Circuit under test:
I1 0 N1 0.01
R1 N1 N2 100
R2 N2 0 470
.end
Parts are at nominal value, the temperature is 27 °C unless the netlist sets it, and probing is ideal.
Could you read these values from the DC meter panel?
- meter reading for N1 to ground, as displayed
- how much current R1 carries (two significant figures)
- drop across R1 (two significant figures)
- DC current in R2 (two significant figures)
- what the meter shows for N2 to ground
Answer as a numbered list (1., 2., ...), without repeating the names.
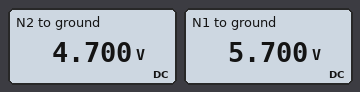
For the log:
1. 5.700 V
2. 10 mA
3. 1.0 V
4. 10 mA
5. 4.700 V
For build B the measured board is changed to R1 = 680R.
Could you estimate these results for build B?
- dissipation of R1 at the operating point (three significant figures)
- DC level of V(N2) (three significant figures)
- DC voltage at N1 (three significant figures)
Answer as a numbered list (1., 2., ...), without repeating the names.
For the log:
1. 68.0 mW
2. 4.70 V
3. 11.5 V
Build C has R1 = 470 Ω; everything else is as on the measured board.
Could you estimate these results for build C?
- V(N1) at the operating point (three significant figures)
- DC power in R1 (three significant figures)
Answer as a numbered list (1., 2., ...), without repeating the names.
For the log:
1. 9.40 V
2. 47.0 mW
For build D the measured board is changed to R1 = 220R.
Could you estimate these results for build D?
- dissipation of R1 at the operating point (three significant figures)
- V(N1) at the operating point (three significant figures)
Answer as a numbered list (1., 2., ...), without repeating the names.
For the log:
1. 22.0 mW
2. 6.90 V
